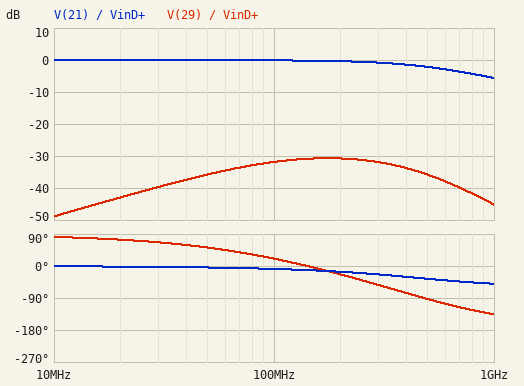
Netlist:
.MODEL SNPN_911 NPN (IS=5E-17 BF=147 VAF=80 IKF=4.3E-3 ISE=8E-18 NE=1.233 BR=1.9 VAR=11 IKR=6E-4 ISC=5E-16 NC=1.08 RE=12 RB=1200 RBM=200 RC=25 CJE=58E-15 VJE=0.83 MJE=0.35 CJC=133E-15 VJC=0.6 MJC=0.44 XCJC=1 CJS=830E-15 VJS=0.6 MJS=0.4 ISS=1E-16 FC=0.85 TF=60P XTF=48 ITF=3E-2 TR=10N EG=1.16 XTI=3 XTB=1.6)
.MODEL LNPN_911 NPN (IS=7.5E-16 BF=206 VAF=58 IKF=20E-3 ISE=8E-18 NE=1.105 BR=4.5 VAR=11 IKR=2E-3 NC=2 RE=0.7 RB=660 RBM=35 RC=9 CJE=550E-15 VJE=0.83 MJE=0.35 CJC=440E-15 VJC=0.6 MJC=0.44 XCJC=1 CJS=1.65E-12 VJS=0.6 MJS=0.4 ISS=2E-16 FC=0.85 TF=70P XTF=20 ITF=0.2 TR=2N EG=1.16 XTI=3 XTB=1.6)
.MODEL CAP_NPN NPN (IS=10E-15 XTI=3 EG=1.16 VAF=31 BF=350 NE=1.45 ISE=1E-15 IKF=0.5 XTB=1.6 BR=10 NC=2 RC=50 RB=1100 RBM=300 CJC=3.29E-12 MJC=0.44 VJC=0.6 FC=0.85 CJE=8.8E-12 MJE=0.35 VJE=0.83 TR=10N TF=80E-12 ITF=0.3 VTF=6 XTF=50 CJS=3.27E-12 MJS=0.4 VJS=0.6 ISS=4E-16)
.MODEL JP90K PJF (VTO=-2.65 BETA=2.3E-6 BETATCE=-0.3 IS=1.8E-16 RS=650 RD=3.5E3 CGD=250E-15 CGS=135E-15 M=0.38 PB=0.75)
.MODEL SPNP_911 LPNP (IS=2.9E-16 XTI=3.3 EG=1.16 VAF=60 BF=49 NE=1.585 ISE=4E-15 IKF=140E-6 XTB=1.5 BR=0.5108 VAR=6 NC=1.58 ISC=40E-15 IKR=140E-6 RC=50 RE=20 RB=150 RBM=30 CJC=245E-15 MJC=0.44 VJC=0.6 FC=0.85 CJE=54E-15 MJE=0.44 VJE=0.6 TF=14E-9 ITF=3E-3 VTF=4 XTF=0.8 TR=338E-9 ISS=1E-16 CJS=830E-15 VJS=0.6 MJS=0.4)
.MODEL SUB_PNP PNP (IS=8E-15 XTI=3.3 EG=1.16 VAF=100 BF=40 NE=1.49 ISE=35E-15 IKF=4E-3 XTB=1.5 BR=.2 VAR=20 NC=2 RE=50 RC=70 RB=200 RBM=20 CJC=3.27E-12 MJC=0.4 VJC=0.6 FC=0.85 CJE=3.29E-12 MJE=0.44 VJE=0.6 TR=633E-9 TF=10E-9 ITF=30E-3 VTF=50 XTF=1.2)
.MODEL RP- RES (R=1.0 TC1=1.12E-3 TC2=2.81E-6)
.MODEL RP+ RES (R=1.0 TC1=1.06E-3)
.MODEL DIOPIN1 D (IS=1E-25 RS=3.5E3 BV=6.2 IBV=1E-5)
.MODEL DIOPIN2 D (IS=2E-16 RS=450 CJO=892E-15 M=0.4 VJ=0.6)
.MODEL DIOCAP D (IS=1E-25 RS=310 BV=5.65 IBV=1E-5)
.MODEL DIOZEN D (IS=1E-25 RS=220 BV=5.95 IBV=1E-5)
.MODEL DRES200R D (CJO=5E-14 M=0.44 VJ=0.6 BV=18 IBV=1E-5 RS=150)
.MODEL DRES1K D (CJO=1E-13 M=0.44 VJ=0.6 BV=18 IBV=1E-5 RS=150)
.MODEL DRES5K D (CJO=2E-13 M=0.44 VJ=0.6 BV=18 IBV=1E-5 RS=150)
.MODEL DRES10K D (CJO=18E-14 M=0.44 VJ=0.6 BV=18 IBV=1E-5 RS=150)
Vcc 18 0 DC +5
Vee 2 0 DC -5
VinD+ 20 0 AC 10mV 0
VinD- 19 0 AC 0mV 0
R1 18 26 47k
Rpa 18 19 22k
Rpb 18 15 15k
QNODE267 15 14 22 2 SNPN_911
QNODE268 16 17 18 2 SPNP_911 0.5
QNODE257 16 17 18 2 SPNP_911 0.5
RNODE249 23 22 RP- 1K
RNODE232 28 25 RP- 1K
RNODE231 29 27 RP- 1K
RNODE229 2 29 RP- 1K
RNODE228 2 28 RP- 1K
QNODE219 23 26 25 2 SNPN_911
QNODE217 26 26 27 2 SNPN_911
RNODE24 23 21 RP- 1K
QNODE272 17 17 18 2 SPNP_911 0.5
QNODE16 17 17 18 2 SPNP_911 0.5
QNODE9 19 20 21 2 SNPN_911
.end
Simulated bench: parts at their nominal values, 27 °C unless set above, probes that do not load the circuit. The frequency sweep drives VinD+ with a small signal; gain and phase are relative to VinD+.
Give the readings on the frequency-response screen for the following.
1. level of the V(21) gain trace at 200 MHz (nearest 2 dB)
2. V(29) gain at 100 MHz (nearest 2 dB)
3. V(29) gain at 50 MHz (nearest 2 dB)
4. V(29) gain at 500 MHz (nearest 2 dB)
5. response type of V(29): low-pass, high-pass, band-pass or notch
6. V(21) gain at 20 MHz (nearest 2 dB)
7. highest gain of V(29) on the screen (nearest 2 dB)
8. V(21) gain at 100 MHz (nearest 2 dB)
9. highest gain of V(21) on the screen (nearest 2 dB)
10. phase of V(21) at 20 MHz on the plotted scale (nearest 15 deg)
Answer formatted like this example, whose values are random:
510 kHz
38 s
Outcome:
0 dB
-32 dB
-36 dB
-36 dB
band-pass
0 dB
-30 dB
0 dB
0 dB
0 deg
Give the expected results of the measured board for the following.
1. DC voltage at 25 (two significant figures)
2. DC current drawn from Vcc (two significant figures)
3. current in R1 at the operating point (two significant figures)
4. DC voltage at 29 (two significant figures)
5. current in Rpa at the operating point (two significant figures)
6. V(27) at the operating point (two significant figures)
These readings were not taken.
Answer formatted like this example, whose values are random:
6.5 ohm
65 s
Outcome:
-4.6 V
420 µA
190 µA
-4.8 V
230 µA
-4.6 V
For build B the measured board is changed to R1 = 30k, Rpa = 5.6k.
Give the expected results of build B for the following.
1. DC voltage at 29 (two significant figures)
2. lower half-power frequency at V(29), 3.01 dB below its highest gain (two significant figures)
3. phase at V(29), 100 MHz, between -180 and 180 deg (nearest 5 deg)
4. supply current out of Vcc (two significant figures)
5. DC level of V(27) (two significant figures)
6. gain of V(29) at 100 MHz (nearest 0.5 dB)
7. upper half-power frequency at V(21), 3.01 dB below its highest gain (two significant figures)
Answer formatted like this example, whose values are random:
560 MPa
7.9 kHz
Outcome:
-4.7 V
73 MHz
25 deg
1.2 mA
-4.4 V
-31.5 dB
670 MHz
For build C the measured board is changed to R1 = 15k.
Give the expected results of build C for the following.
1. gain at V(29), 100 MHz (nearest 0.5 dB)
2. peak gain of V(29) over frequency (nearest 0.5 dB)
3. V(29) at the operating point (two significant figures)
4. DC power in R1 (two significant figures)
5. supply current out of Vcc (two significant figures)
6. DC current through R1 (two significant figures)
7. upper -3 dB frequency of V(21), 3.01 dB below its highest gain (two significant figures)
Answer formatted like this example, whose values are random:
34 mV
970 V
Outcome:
-30.5 dB
-28.5 dB
-4.5 V
4.4 mW
770 µA
540 µA
730 MHz
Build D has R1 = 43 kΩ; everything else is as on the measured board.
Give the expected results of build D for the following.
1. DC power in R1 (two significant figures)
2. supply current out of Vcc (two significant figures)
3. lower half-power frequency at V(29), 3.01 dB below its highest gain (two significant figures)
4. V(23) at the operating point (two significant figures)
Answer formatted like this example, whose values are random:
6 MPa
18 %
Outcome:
1.8 mW
430 µA
70 MHz
-960 mV
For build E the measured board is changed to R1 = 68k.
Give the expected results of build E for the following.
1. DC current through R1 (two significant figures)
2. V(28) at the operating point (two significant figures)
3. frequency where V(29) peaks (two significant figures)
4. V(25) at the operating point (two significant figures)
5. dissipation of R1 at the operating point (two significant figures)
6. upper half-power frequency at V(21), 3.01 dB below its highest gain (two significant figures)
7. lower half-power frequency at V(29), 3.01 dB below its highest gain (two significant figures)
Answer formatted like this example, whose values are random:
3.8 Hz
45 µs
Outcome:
130 µA
-4.9 V
170 MHz
-4.7 V
1.2 mW
560 MHz
65 MHz
